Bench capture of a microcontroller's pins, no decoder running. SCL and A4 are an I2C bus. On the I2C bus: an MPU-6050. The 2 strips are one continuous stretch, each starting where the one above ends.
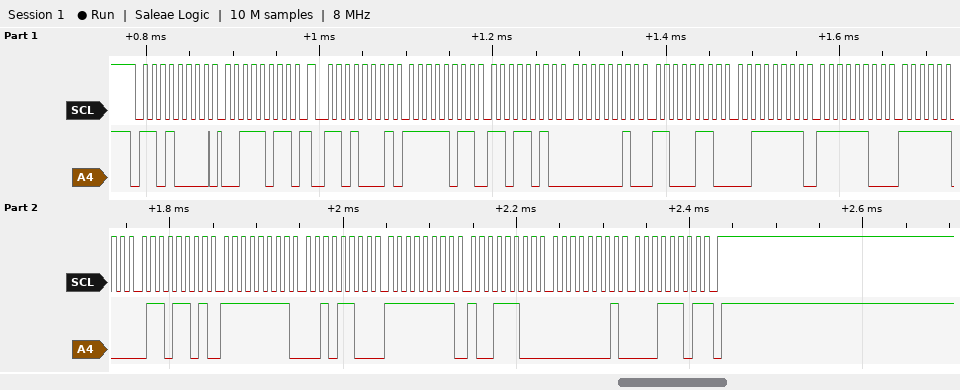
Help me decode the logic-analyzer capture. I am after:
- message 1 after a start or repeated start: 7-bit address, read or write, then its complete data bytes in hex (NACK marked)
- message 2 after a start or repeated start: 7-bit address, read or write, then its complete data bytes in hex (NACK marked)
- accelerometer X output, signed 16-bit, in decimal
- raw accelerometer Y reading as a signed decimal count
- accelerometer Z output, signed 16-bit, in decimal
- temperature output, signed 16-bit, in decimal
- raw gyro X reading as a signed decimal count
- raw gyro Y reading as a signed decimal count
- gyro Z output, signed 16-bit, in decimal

0x68 write: 3B
0x68 read: FB DA 02 C6 3F FC FC 6D FF 2C FF 9C 01 1D NACK
-1062
710
16380
-915
-212
-100
285
